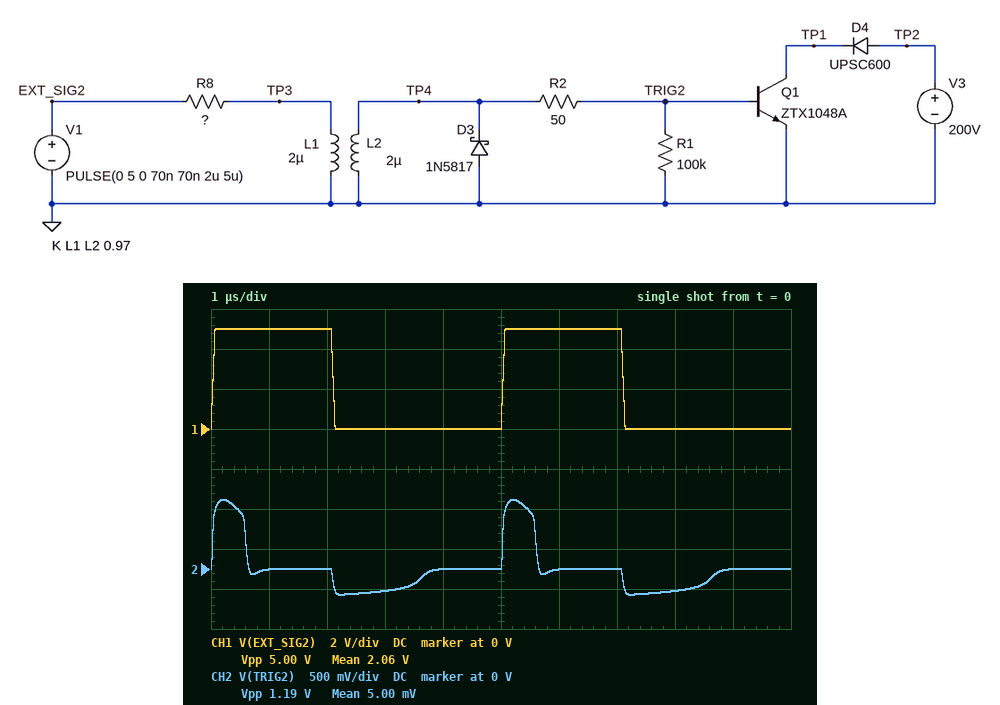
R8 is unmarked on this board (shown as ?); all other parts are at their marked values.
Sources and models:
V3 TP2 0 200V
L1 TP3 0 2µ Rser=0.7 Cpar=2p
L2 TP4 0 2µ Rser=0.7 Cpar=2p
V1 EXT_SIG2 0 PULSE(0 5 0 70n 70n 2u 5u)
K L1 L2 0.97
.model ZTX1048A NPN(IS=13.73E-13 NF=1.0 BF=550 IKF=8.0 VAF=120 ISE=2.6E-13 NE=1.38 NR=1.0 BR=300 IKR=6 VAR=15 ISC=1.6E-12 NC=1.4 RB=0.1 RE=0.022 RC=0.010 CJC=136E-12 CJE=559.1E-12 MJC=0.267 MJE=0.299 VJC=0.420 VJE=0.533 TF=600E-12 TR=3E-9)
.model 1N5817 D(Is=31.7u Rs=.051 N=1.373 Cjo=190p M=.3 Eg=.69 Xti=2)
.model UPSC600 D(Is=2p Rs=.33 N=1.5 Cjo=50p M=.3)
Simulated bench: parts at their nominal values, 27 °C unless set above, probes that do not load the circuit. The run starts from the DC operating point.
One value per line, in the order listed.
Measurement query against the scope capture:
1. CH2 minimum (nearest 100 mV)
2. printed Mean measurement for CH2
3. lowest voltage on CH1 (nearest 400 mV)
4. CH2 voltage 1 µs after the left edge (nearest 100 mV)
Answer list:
-300 mV
5.00 mV
0 V
0 V
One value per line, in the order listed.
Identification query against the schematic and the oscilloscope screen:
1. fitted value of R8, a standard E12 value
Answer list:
18 Ω
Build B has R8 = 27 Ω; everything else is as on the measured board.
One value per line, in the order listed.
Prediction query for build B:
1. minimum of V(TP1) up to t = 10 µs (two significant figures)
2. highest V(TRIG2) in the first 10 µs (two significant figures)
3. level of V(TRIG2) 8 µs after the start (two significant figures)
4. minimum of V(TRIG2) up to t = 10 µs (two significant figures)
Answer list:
200 V
810 mV
-230 mV
-300 mV
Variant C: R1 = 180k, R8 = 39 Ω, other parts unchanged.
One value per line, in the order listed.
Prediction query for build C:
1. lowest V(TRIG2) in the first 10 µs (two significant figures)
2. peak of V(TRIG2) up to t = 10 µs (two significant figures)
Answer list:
-290 mV
760 mV
